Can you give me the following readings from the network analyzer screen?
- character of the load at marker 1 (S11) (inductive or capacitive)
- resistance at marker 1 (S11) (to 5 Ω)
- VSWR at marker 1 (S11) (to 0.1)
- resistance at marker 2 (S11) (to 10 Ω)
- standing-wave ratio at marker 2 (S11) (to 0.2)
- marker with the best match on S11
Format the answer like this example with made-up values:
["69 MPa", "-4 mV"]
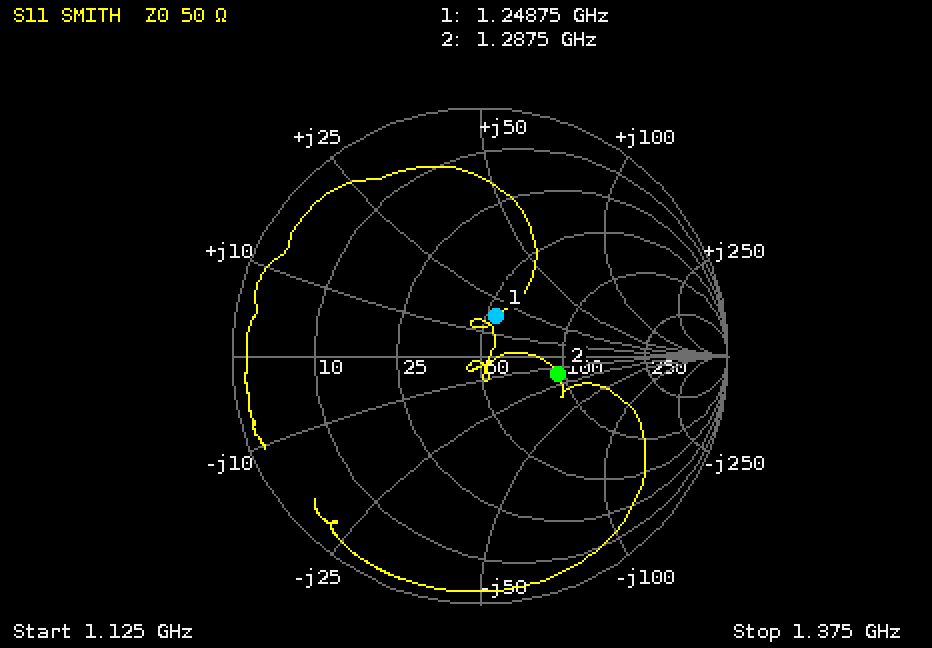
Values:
["inductive", "55 Ω", "1.4", "90 Ω", "2.0", "marker 1"]
